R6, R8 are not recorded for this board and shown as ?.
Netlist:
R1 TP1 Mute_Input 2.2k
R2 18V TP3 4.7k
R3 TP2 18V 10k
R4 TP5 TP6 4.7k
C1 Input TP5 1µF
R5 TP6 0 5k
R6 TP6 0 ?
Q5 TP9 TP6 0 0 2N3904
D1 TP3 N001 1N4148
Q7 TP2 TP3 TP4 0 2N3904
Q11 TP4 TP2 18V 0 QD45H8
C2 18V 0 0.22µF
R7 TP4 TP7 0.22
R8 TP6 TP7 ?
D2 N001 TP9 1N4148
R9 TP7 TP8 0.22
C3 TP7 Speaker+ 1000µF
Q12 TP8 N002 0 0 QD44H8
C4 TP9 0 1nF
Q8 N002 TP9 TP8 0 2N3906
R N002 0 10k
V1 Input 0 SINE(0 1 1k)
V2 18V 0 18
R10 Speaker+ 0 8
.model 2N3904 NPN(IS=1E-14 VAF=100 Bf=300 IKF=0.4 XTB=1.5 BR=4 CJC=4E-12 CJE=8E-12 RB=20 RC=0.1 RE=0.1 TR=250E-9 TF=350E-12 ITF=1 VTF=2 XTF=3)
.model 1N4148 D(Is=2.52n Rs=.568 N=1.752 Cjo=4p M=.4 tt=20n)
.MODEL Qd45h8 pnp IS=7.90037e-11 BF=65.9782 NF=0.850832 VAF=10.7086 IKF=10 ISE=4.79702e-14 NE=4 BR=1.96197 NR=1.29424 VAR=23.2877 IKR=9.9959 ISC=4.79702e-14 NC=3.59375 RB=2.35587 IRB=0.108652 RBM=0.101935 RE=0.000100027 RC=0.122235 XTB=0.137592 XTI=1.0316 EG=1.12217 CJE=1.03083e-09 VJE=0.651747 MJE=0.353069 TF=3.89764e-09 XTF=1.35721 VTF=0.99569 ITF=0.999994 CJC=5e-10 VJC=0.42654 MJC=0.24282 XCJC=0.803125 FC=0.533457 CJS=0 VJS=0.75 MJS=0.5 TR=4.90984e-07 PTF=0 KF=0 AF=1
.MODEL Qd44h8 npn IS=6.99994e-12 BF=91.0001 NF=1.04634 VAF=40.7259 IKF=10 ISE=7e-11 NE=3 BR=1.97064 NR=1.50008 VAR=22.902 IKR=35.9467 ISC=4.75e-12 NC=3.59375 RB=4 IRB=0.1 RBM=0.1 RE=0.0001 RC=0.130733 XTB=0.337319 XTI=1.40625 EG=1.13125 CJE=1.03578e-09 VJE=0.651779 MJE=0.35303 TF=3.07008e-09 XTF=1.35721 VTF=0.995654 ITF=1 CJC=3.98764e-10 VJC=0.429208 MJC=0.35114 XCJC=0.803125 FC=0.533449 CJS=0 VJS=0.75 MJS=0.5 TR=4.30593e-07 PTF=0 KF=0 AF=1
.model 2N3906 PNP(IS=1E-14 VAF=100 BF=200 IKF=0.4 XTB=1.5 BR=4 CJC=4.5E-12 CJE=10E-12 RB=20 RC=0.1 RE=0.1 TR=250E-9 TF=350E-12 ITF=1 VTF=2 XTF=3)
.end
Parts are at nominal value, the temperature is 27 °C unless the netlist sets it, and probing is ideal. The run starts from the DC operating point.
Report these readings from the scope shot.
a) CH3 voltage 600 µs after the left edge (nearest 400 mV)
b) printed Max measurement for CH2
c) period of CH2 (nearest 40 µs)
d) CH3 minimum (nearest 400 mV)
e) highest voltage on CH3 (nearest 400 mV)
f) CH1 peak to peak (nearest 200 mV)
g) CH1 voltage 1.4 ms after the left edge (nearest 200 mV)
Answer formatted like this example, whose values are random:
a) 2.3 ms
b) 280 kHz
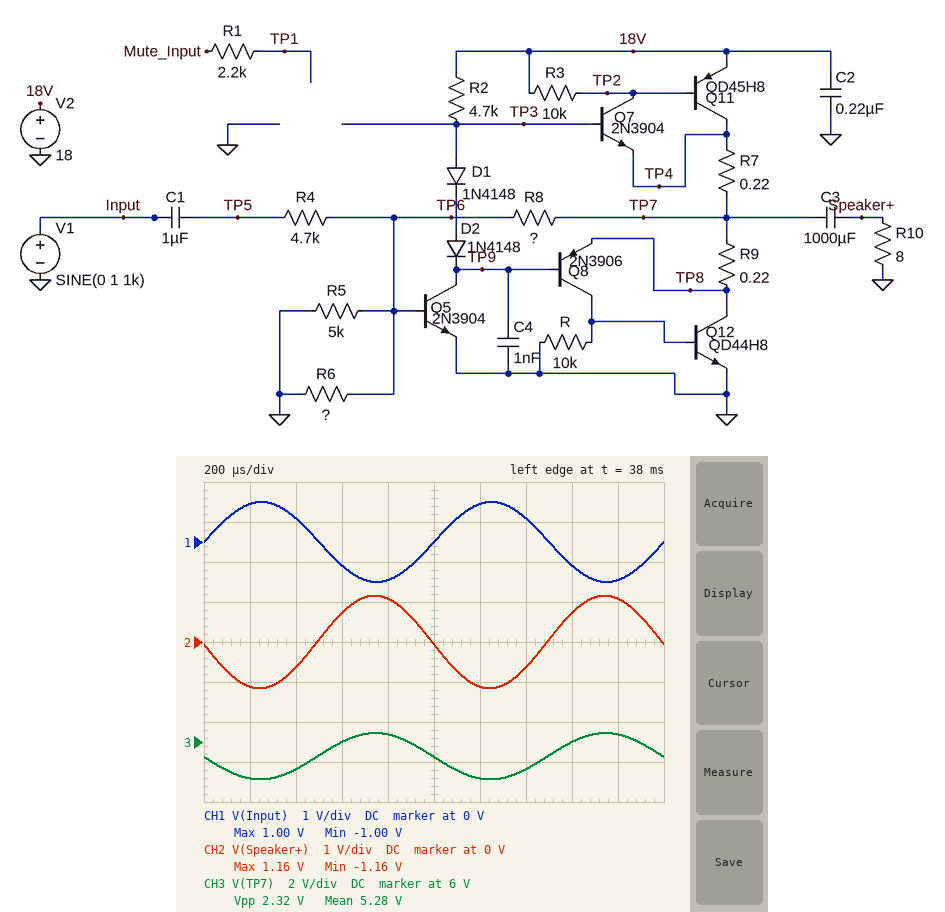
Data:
a) 6.0 V
b) 1.16 V
c) 1.00 ms
d) 4.0 V
e) 6.4 V
f) 2.0 V
g) 600 mV
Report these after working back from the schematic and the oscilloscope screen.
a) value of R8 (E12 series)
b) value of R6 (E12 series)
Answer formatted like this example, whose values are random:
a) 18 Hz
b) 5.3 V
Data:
a) 5.6 kΩ
b) 1 kΩ
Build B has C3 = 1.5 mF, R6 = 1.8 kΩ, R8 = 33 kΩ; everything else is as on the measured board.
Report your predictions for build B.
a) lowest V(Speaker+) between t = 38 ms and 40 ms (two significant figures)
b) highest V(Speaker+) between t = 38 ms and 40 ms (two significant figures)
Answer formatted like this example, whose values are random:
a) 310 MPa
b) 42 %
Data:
a) -3.5 V
b) 2.7 V
